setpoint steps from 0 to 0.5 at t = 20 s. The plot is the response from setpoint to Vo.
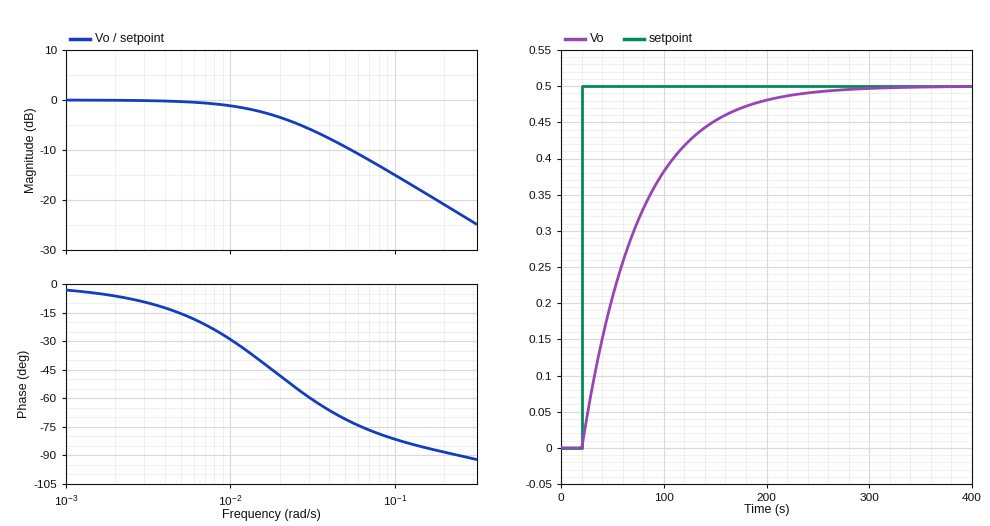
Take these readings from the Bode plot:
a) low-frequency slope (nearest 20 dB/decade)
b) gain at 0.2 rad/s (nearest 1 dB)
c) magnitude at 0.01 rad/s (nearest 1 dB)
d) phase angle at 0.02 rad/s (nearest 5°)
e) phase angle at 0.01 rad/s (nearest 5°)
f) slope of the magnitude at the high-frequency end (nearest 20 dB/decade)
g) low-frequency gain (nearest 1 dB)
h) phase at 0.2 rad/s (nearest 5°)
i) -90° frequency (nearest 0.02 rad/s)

0 dB/decade
-21 dB
-1 dB
-50°
-30°
-20 dB/decade
0 dB
-90°
0.24 rad/s
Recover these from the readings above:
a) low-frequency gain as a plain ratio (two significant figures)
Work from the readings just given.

1.0
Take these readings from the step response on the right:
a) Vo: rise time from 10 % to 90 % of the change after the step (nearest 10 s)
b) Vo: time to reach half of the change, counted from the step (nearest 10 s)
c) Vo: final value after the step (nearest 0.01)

120 s
40 s
0.50
